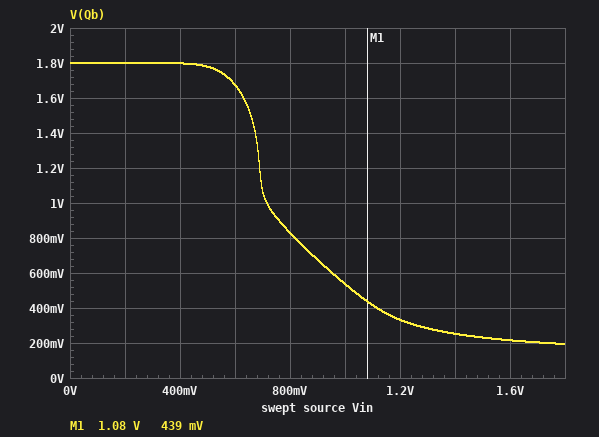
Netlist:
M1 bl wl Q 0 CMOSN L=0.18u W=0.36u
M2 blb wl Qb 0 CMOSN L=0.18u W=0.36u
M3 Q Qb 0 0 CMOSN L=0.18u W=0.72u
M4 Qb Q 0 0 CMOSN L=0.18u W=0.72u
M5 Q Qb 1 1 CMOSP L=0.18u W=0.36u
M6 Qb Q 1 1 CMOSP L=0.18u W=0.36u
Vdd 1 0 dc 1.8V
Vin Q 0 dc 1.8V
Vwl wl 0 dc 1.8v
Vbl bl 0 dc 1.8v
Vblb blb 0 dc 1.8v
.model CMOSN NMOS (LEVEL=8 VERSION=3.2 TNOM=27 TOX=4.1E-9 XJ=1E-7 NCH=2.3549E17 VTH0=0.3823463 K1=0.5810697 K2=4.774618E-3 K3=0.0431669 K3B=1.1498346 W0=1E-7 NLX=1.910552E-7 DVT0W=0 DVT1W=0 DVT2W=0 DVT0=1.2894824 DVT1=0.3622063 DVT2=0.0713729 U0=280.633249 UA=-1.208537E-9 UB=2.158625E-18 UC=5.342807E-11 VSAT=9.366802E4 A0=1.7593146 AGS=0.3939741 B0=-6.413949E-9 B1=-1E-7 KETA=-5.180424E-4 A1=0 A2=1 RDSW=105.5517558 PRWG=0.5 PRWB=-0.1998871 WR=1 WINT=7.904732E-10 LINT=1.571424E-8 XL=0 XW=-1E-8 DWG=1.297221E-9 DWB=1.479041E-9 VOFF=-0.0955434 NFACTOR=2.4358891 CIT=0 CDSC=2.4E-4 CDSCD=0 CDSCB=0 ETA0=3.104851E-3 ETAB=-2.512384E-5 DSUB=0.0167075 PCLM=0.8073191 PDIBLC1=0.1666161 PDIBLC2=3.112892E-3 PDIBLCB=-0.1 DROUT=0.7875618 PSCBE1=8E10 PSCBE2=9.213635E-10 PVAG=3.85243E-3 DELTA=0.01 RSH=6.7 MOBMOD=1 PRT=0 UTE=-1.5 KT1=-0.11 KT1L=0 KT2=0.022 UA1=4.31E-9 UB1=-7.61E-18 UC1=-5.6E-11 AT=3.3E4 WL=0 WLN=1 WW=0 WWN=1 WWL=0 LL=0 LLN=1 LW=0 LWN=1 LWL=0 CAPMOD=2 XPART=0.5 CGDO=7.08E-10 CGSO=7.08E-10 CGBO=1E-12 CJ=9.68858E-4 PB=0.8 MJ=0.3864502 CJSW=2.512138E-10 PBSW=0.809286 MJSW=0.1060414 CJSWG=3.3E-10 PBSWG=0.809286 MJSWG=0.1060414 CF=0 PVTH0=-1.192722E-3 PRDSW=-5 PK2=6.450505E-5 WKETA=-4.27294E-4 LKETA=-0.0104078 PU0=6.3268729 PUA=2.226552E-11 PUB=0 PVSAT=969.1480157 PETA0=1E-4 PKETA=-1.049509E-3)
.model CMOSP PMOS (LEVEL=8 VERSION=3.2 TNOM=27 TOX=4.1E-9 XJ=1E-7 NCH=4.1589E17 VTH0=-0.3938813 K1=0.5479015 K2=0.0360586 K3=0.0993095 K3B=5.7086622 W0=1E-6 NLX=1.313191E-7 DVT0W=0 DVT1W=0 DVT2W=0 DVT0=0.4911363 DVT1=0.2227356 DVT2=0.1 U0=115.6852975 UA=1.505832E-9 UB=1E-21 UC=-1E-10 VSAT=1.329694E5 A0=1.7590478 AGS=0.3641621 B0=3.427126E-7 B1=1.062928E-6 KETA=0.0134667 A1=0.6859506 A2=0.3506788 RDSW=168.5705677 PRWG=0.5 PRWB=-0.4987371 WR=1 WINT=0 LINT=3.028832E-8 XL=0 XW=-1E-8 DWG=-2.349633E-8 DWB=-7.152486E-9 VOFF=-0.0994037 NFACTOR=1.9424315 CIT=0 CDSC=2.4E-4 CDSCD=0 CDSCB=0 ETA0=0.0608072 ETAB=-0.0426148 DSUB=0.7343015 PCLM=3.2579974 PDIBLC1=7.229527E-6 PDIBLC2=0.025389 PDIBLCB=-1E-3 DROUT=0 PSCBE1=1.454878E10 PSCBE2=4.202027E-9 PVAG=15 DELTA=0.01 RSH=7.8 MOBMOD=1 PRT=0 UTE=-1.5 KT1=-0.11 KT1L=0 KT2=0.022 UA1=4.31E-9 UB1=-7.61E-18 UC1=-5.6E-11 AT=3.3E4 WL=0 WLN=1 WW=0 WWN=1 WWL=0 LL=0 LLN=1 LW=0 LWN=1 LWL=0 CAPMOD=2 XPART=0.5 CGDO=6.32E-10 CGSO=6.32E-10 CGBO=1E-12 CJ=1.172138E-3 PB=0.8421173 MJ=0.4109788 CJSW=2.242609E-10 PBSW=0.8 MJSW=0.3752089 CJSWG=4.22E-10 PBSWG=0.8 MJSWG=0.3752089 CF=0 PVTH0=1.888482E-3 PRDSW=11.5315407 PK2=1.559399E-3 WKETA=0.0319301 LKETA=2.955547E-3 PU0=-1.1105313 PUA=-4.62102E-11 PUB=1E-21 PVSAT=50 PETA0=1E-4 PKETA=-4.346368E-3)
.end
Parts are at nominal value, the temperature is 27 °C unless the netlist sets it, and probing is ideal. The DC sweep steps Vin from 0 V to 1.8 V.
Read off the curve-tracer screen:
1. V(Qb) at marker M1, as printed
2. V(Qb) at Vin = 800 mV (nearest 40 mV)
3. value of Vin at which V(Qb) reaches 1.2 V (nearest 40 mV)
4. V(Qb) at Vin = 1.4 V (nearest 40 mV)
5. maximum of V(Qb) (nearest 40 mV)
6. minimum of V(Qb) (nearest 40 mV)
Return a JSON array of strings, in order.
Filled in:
["439 mV", "840 mV", "680 mV", "240 mV", "1.80 V", "200 mV"]
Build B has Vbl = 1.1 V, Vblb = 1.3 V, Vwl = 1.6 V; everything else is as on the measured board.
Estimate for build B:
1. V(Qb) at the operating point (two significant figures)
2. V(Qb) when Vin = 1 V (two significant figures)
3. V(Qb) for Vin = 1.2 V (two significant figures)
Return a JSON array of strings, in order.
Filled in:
["150 mV", "380 mV", "240 mV"]
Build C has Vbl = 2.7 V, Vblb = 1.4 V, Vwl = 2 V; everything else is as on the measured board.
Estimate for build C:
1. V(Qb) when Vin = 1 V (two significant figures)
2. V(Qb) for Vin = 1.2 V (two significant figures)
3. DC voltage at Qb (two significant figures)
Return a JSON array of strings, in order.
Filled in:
["660 mV", "420 mV", "230 mV"]
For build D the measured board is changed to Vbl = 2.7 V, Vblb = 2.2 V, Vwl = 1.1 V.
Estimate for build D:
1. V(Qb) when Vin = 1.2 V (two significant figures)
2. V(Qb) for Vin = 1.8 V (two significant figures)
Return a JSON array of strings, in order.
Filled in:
["110 mV", "71 mV"]
